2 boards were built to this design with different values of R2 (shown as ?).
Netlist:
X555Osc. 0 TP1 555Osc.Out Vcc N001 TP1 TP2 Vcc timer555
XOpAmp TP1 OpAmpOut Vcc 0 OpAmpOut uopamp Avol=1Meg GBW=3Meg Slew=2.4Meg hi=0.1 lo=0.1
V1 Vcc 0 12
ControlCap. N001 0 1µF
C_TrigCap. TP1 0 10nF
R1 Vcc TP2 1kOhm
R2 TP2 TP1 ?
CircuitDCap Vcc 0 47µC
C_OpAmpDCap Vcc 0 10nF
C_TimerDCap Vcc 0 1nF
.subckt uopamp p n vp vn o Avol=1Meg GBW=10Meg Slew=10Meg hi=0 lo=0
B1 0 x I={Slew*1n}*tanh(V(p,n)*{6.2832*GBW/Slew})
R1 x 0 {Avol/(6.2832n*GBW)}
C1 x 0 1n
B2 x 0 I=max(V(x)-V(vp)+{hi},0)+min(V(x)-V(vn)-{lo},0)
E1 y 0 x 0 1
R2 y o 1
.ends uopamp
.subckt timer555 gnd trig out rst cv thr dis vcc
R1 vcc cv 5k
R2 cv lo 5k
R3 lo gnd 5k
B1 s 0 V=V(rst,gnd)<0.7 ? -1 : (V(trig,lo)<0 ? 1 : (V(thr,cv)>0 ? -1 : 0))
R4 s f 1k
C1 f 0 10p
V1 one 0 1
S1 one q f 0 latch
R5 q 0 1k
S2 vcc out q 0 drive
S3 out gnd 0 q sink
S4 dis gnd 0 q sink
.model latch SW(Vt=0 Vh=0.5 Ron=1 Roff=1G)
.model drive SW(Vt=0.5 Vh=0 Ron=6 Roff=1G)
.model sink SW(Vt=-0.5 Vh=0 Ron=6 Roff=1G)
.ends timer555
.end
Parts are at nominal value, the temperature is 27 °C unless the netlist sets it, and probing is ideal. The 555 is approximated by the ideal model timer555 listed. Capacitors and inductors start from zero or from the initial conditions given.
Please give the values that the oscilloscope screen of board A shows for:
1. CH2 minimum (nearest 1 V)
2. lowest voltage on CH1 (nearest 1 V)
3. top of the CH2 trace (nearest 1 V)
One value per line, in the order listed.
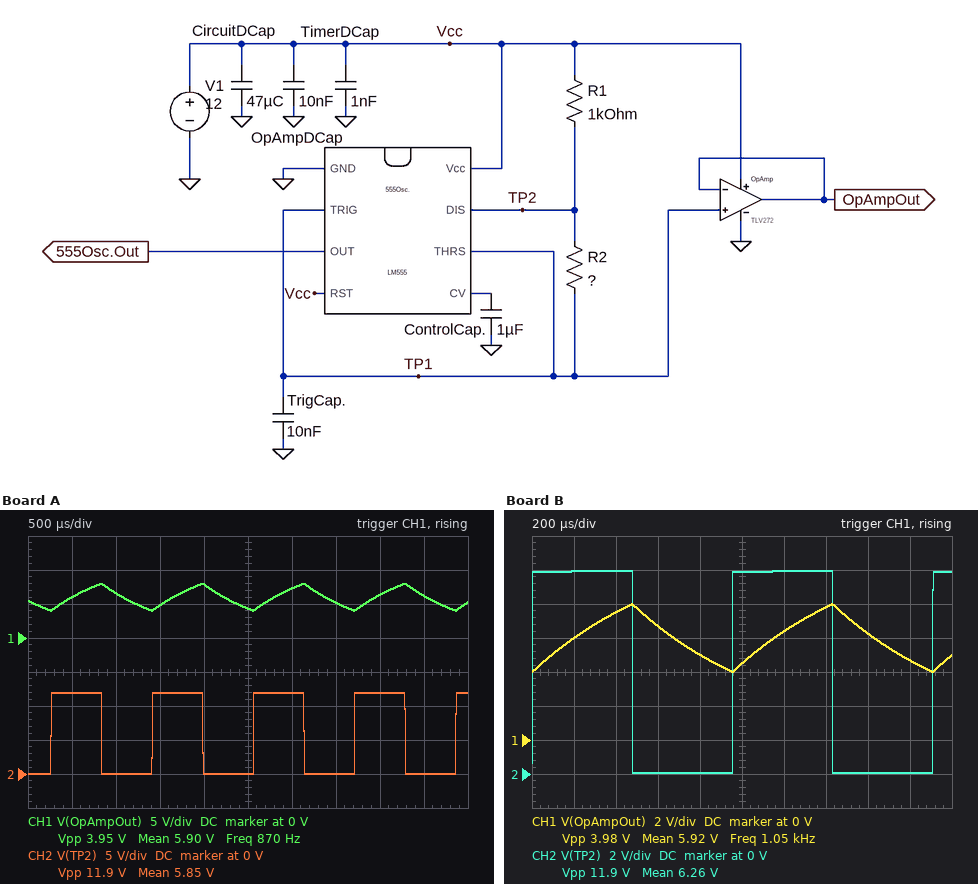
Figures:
0 V
4 V
12 V
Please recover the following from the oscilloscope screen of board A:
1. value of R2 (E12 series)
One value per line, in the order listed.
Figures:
82 kΩ
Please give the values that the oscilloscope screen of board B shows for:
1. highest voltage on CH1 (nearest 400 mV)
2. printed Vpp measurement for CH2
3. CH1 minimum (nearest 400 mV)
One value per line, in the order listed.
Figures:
8.0 V
11.9 V
4.0 V
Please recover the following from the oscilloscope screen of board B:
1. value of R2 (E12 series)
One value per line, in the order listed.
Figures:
68 kΩ
